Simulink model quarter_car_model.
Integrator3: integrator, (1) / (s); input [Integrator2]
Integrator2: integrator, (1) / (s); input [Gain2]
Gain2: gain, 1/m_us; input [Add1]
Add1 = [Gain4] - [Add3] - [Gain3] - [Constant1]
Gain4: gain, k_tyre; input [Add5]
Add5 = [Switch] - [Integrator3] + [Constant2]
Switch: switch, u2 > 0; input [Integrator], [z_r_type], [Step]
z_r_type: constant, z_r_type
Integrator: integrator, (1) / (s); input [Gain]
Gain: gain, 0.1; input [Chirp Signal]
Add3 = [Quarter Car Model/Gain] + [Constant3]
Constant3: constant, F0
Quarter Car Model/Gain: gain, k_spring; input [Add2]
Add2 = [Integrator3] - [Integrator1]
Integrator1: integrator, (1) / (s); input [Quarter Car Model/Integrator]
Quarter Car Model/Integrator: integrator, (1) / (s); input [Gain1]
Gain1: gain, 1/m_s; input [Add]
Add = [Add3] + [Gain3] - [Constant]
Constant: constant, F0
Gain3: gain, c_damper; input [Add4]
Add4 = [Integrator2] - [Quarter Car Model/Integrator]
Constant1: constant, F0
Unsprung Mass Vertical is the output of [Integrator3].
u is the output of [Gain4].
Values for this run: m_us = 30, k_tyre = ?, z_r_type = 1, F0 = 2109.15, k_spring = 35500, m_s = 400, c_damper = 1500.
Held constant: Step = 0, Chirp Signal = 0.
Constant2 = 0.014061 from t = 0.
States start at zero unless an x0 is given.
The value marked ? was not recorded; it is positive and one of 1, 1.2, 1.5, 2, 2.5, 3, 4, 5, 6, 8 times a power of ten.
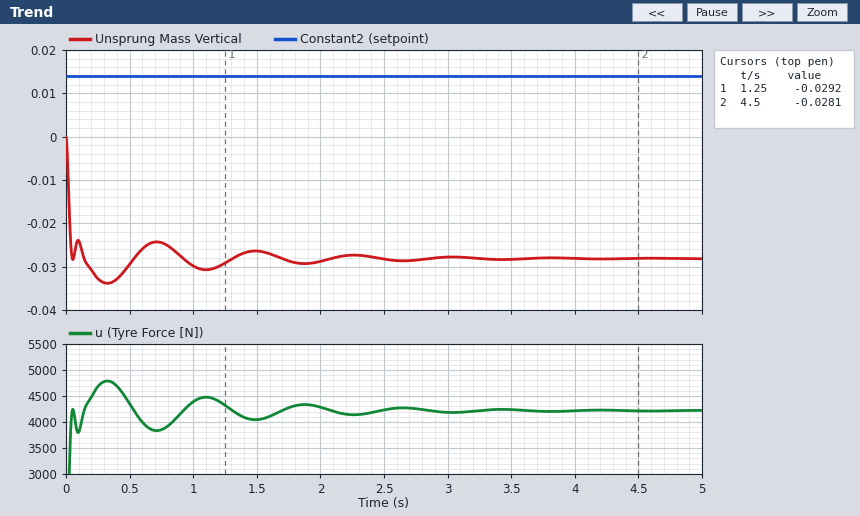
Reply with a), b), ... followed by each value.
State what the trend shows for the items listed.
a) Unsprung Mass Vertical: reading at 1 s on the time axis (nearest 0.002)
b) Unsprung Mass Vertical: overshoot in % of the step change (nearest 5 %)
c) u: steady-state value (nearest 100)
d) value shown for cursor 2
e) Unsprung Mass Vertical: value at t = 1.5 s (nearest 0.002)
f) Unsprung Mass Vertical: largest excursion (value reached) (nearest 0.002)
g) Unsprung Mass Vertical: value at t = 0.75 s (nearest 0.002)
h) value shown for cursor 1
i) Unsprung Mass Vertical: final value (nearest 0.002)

a) -0.030
b) 20 %
c) 4200
d) -0.0281
e) -0.026
f) -0.034
g) -0.024
h) -0.0292
i) -0.028
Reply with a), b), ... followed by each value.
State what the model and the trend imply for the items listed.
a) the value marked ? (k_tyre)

a) 100000
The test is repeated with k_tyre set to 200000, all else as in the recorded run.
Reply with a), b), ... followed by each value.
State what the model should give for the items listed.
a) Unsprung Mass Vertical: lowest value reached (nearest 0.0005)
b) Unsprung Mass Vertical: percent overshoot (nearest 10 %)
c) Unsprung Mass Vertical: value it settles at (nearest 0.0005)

a) -0.0085
b) 20 %
c) -0.0070
